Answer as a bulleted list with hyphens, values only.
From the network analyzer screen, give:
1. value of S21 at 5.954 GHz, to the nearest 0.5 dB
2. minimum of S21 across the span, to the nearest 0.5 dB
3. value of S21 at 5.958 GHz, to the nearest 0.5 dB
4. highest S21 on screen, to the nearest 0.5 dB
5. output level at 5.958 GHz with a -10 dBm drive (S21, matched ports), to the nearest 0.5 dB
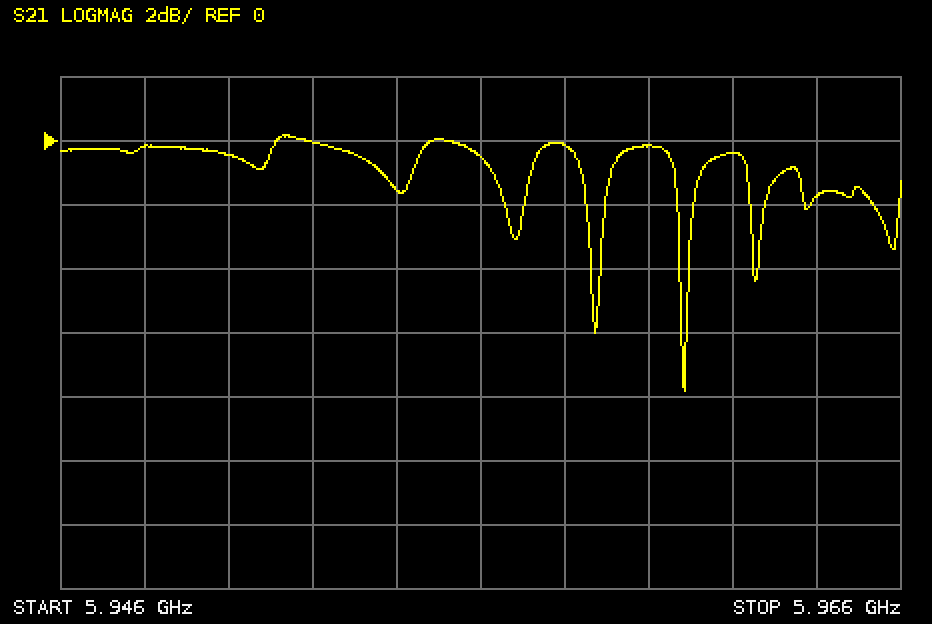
- -1.5 dB
- -8.0 dB
- 0.0 dB
- 0.0 dB
- -10.0 dBm
